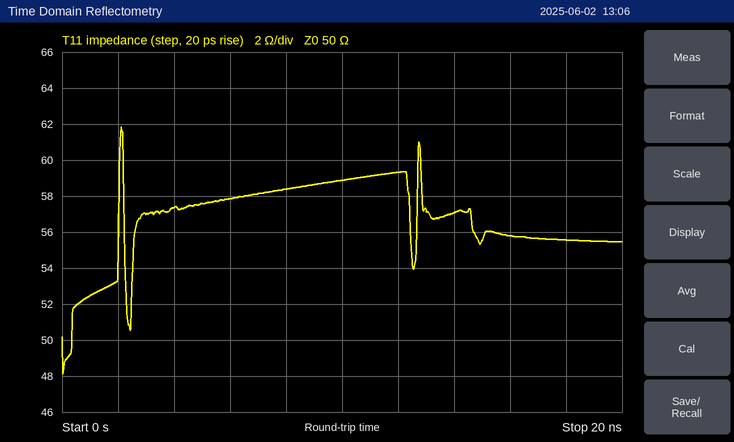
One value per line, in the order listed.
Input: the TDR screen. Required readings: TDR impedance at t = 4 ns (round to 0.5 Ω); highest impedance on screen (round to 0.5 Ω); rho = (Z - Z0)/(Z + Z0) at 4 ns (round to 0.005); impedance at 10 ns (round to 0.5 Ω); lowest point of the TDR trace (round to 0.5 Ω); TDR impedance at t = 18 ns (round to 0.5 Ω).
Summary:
57.5 Ω
62.0 Ω
+0.070
59.0 Ω
48.0 Ω
55.5 Ω
